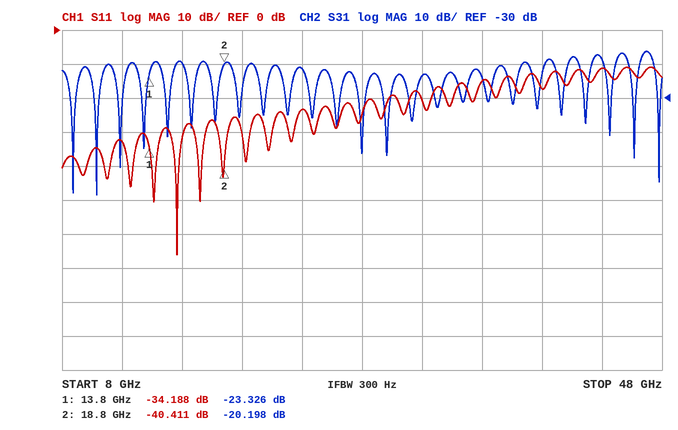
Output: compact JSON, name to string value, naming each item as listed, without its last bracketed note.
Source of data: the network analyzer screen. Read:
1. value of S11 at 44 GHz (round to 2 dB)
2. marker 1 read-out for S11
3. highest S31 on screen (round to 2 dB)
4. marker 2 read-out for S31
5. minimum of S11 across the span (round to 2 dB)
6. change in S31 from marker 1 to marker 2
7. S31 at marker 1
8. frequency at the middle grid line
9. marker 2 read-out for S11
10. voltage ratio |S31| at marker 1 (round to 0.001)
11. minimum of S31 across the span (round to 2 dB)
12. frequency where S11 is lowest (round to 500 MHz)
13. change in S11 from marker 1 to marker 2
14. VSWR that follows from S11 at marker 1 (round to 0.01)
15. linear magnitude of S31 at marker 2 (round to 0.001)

{"value of S11 at 44 GHz": "-12 dB", "marker 1 read-out for S11": "-34.188 dB", "highest S31 on screen": "-16 dB", "marker 2 read-out for S31": "-20.198 dB", "minimum of S11 across the span": "-66 dB", "change in S31 from marker 1 to marker 2": "3.128 dB", "S31 at marker 1": "-23.326 dB", "frequency at the middle grid line": "28 GHz", "marker 2 read-out for S11": "-40.411 dB", "voltage ratio |S31| at marker 1": "0.068", "minimum of S31 across the span": "-58 dB", "frequency where S11 is lowest": "15.5 GHz", "change in S11 from marker 1 to marker 2": "-6.223 dB", "VSWR that follows from S11 at marker 1": "1.04", "linear magnitude of S31 at marker 2": "0.098"}
